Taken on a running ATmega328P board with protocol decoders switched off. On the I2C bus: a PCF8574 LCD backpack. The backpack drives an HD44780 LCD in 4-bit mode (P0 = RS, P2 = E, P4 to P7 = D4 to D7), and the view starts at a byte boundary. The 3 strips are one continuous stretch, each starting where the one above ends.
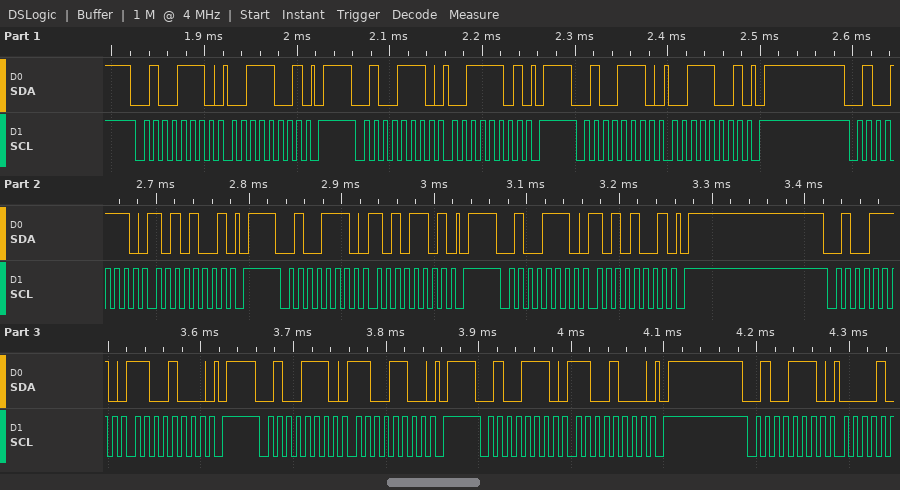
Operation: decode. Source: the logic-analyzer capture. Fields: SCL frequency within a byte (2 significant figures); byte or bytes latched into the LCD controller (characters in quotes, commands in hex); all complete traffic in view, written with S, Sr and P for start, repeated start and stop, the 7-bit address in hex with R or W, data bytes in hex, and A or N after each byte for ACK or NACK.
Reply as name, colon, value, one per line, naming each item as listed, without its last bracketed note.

SCL frequency within a byte: 100 kHz
byte or bytes latched into the LCD controller: ':'
all complete traffic in view, written with S, Sr and P for start, repeated start and stop, the 7-bit address in hex with R or W, data bytes in hex, and A or N after each byte for ACK or NACK: S 27W A 39 A P S 27W A 3D A P S 27W A 39 A P S 27W A A9 A P S 27W A AD A P S 27W A A9 A P S 27W A C8 A P S 27W A CC A P S 27W A C8 A P S 27W A
